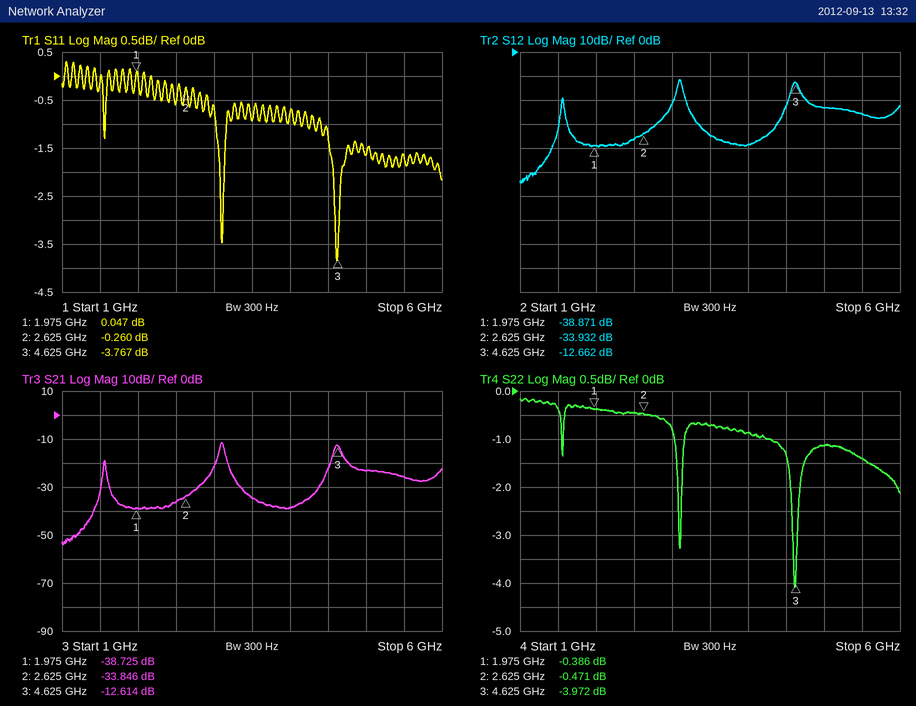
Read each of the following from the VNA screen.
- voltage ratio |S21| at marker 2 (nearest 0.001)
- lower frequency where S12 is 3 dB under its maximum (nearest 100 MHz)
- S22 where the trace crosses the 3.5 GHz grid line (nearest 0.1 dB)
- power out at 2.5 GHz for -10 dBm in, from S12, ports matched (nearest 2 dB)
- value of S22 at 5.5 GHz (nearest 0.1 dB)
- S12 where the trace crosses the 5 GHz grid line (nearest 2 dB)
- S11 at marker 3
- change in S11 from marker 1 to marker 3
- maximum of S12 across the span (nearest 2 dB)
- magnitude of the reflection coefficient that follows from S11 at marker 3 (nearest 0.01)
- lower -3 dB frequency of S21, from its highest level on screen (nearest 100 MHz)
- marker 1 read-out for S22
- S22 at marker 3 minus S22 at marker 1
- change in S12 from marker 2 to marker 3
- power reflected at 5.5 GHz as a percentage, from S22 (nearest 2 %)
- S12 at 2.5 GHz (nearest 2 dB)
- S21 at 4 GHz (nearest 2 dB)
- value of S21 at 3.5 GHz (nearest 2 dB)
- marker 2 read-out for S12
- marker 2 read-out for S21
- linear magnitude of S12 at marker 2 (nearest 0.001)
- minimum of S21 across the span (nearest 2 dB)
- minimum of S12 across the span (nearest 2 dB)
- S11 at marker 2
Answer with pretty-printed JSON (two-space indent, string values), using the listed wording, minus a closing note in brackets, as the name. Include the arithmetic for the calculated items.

{
  "voltage ratio |S21| at marker 2": "10^(-33.846/20) ≈ 0.020",
  "lower frequency where S12 is 3 dB under its maximum": "3.1 GHz",
  "S22 where the trace crosses the 3.5 GHz grid line": "-0.7 dB",
  "power out at 2.5 GHz for -10 dBm in, from S12, ports matched": "-10 dBm + (-36 dB) = -46 dBm",
  "value of S22 at 5.5 GHz": "-1.4 dB",
  "S12 where the trace crosses the 5 GHz grid line": "-24 dB",
  "S11 at marker 3": "-3.767 dB",
  "change in S11 from marker 1 to marker 3": "-3.767 − (0.047) = -3.814 dB",
  "maximum of S12 across the span": "-12 dB",
  "magnitude of the reflection coefficient that follows from S11 at marker 3": "10^(-3.767/20) ≈ 0.65",
  "lower -3 dB frequency of S21, from its highest level on screen": "3.1 GHz",
  "marker 1 read-out for S22": "-0.386 dB",
  "S22 at marker 3 minus S22 at marker 1": "-3.972 − (-0.386) = -3.586 dB",
  "change in S12 from marker 2 to marker 3": "-12.662 − (-33.932) = 21.270 dB",
  "power reflected at 5.5 GHz as a percentage, from S22": "10^(-1.4/10) ≈ 72 %",
  "S12 at 2.5 GHz": "-36 dB",
  "S21 at 4 GHz": "-38 dB",
  "value of S21 at 3.5 GHz": "-34 dB",
  "marker 2 read-out for S12": "-33.932 dB",
  "marker 2 read-out for S21": "-33.846 dB",
  "linear magnitude of S12 at marker 2": "10^(-33.932/20) ≈ 0.020",
  "minimum of S21 across the span": "-54 dB",
  "minimum of S12 across the span": "-54 dB",
  "S11 at marker 2": "-0.260 dB"
}
